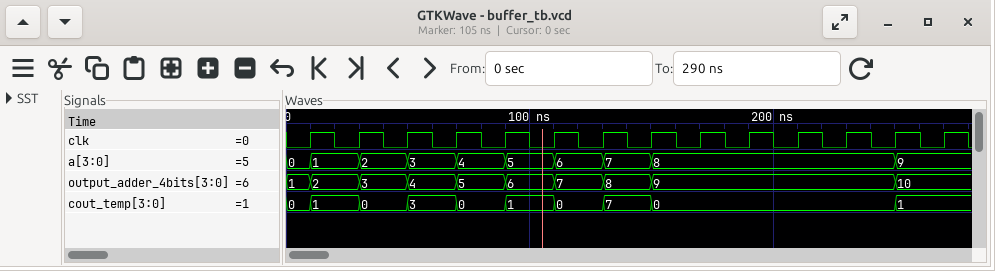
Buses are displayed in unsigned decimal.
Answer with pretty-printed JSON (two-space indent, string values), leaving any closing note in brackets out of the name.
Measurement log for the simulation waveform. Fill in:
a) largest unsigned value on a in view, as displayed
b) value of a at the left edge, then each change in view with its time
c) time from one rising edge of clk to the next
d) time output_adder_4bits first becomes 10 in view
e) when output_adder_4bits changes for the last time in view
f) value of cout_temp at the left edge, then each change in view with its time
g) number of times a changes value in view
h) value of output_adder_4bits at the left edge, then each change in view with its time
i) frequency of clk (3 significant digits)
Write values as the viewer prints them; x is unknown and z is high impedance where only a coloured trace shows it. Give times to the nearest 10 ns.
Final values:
{
  "largest unsigned value on a in view, as displayed": "9",
  "value of a at the left edge, then each change in view with its time": "0, 1 at 10 ns, 2 at 30 ns, 3 at 50 ns, 4 at 70 ns, 5 at 90 ns, 6 at 110 ns, 7 at 130 ns, 8 at 150 ns, 9 at 250 ns",
  "time from one rising edge of clk to the next": "20 ns",
  "time output_adder_4bits first becomes 10 in view": "250 ns",
  "when output_adder_4bits changes for the last time in view": "250 ns",
  "value of cout_temp at the left edge, then each change in view with its time": "0, 1 at 10 ns, 0 at 30 ns, 3 at 50 ns, 0 at 70 ns, 1 at 90 ns, 0 at 110 ns, 7 at 130 ns, 0 at 150 ns, 1 at 250 ns",
  "number of times a changes value in view": "9",
  "value of output_adder_4bits at the left edge, then each change in view with its time": "1, 2 at 10 ns, 3 at 30 ns, 4 at 50 ns, 5 at 70 ns, 6 at 90 ns, 7 at 110 ns, 8 at 130 ns, 9 at 150 ns, 10 at 250 ns",
  "frequency of clk": "50.0 MHz"
}
